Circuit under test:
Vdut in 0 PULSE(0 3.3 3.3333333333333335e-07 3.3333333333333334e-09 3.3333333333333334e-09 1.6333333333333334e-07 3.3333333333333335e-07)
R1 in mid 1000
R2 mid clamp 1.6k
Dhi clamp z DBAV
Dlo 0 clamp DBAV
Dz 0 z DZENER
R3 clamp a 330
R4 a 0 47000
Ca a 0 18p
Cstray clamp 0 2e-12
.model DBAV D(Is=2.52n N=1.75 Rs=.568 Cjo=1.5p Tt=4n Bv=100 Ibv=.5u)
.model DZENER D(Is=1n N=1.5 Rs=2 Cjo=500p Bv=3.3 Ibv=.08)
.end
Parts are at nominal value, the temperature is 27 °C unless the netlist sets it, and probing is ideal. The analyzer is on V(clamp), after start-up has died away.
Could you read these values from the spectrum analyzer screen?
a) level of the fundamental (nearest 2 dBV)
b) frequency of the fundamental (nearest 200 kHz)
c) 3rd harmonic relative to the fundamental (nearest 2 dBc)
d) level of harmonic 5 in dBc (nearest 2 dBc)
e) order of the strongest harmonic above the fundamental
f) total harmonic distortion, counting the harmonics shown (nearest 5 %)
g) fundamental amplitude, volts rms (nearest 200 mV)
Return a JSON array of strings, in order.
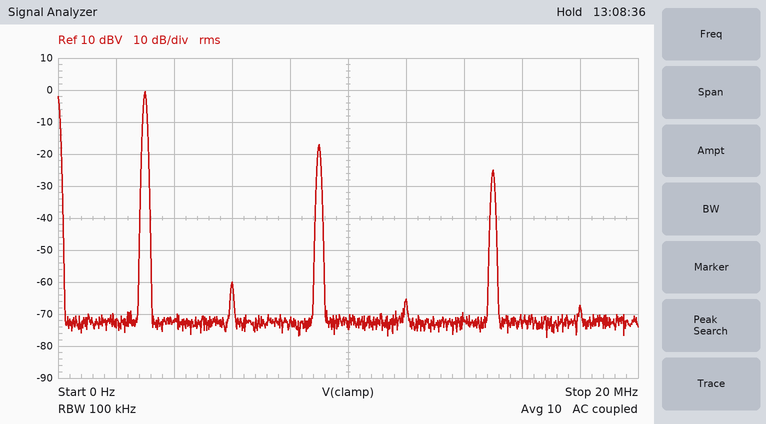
["0 dBV", "3.0 MHz", "-16 dBc", "-24 dBc", "3", "15 %", "1.0 V"]
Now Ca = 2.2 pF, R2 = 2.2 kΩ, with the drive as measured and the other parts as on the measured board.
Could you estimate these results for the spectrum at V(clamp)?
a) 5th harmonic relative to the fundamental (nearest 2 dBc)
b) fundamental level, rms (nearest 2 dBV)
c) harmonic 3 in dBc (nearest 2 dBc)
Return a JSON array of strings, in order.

["-20 dBc", "2 dBV", "-12 dBc"]
